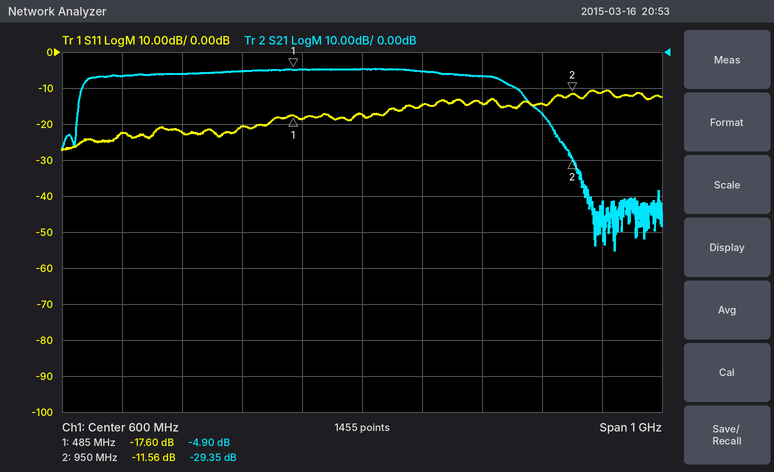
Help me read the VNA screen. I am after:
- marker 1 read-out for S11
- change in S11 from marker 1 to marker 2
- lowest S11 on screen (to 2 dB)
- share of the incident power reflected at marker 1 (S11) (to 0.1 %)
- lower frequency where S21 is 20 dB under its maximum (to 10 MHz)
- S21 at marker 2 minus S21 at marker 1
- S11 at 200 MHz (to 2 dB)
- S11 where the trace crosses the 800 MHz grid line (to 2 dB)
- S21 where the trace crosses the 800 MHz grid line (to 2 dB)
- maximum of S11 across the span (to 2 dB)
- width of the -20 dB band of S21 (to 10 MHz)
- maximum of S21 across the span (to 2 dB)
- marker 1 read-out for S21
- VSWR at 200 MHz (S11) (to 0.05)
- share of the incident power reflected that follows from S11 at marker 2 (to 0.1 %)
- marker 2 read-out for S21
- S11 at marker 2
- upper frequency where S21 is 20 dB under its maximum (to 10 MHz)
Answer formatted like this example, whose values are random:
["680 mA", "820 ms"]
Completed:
["-17.60 dB", "6.04 dB", "-28 dB", "1.7 %", "120 MHz", "-24.45 dB", "-22 dB", "-14 dB", "-6 dB", "-10 dB", "810 MHz", "-4 dB", "-4.90 dB", "1.15", "7.0 %", "-29.35 dB", "-11.56 dB", "930 MHz"]
